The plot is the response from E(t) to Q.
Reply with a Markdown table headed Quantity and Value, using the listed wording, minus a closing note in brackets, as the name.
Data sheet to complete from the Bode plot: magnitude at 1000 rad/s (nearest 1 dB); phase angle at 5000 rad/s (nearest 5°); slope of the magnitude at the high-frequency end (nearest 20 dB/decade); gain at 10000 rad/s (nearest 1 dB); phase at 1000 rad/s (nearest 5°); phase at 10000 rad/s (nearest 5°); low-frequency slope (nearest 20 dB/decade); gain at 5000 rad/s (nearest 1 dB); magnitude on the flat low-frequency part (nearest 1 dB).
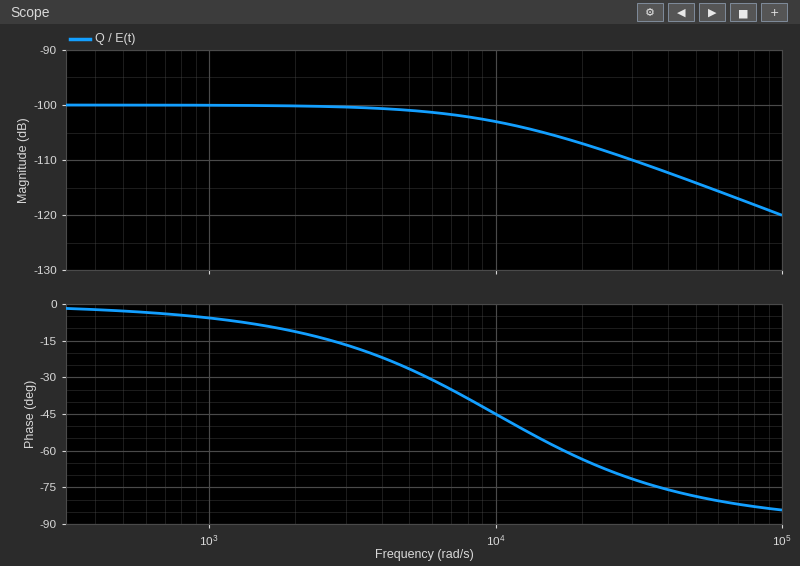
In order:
| Quantity | Value |
|---|---|
| magnitude at 1000 rad/s | -100 dB |
| phase angle at 5000 rad/s | -25° |
| slope of the magnitude at the high-frequency end | -20 dB/decade |
| gain at 10000 rad/s | -103 dB |
| phase at 1000 rad/s | -5° |
| phase at 10000 rad/s | -45° |
| low-frequency slope | 0 dB/decade |
| gain at 5000 rad/s | -101 dB |
| magnitude on the flat low-frequency part | -100 dB |
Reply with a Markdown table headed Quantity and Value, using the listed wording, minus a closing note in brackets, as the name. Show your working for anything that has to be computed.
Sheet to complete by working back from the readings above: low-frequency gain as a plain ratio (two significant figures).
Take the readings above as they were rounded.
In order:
| Quantity | Value |
|---|---|
| low-frequency gain as a plain ratio | 10^(-100 / 20) = 0.000010 |
